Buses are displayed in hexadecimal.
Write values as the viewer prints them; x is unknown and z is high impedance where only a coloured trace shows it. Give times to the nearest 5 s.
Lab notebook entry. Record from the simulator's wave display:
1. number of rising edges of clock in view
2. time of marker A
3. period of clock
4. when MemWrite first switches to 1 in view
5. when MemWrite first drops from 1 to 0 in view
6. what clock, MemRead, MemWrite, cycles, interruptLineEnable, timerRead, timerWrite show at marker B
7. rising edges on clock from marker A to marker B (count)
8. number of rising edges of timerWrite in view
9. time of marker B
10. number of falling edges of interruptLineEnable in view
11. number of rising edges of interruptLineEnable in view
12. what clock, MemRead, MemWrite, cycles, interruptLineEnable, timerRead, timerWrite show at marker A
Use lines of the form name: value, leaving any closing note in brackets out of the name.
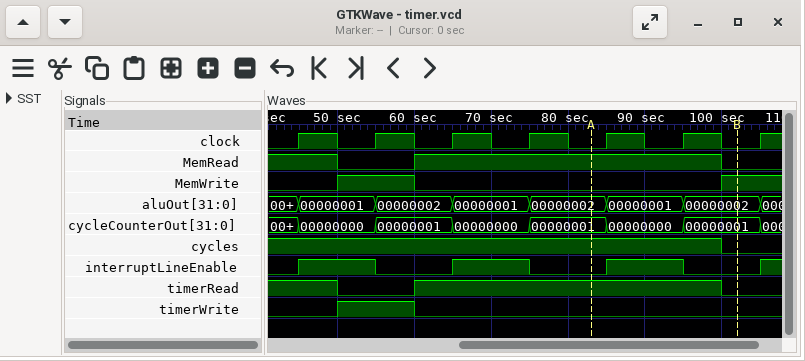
number of rising edges of clock in view: 7
time of marker A: 85 s
period of clock: 10 s
when MemWrite first switches to 1 in view: 50 s
when MemWrite first drops from 1 to 0 in view: 60 s
what clock, MemRead, MemWrite, cycles, interruptLineEnable, timerRead, timerWrite show at marker B: clock=0, MemRead=0, MemWrite=1, cycles=0, interruptLineEnable=0, timerRead=0, timerWrite=0
rising edges on clock from marker A to marker B: 2
number of rising edges of timerWrite in view: 1
time of marker B: 100 s
number of falling edges of interruptLineEnable in view: 3
number of rising edges of interruptLineEnable in view: 4
what clock, MemRead, MemWrite, cycles, interruptLineEnable, timerRead, timerWrite show at marker A: clock=0, MemRead=1, MemWrite=0, cycles=1, interruptLineEnable=0, timerRead=1, timerWrite=0
